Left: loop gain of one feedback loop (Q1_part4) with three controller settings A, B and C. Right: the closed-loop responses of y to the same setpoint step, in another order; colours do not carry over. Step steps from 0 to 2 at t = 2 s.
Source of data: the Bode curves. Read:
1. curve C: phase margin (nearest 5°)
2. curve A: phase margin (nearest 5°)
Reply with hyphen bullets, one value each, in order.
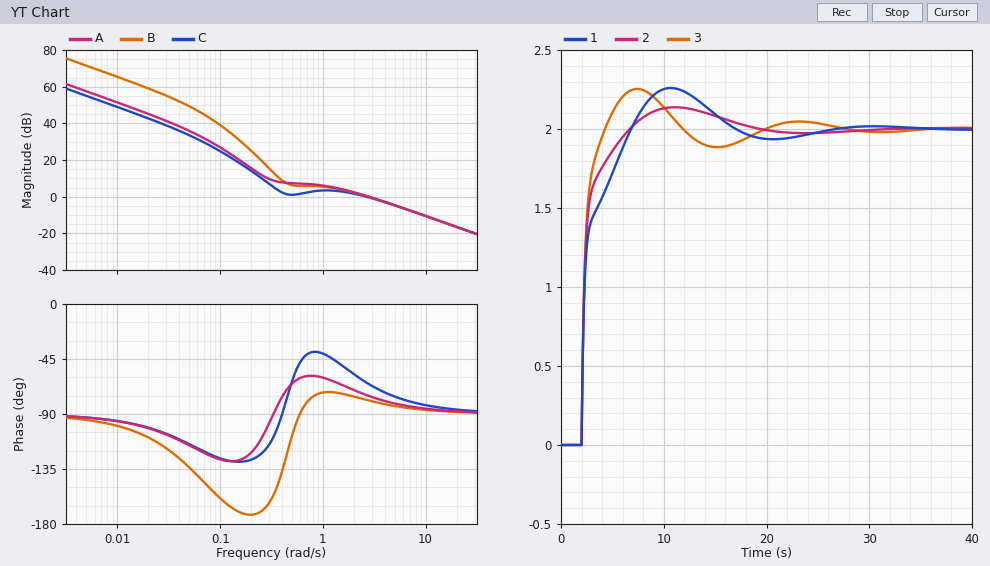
- 115°
- 105°
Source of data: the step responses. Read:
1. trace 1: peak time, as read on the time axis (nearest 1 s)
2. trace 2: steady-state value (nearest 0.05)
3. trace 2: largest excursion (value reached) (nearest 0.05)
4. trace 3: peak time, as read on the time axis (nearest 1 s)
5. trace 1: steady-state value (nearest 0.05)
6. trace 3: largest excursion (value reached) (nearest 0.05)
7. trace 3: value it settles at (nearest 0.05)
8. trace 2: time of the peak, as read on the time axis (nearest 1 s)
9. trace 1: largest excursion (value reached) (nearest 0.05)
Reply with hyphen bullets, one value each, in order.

- 11 s
- 2.00
- 2.15
- 7 s
- 2.00
- 2.25
- 2.00
- 11 s
- 2.25
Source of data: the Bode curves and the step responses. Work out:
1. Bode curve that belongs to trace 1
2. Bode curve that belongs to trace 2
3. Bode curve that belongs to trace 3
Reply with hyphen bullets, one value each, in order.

- C
- A
- B
